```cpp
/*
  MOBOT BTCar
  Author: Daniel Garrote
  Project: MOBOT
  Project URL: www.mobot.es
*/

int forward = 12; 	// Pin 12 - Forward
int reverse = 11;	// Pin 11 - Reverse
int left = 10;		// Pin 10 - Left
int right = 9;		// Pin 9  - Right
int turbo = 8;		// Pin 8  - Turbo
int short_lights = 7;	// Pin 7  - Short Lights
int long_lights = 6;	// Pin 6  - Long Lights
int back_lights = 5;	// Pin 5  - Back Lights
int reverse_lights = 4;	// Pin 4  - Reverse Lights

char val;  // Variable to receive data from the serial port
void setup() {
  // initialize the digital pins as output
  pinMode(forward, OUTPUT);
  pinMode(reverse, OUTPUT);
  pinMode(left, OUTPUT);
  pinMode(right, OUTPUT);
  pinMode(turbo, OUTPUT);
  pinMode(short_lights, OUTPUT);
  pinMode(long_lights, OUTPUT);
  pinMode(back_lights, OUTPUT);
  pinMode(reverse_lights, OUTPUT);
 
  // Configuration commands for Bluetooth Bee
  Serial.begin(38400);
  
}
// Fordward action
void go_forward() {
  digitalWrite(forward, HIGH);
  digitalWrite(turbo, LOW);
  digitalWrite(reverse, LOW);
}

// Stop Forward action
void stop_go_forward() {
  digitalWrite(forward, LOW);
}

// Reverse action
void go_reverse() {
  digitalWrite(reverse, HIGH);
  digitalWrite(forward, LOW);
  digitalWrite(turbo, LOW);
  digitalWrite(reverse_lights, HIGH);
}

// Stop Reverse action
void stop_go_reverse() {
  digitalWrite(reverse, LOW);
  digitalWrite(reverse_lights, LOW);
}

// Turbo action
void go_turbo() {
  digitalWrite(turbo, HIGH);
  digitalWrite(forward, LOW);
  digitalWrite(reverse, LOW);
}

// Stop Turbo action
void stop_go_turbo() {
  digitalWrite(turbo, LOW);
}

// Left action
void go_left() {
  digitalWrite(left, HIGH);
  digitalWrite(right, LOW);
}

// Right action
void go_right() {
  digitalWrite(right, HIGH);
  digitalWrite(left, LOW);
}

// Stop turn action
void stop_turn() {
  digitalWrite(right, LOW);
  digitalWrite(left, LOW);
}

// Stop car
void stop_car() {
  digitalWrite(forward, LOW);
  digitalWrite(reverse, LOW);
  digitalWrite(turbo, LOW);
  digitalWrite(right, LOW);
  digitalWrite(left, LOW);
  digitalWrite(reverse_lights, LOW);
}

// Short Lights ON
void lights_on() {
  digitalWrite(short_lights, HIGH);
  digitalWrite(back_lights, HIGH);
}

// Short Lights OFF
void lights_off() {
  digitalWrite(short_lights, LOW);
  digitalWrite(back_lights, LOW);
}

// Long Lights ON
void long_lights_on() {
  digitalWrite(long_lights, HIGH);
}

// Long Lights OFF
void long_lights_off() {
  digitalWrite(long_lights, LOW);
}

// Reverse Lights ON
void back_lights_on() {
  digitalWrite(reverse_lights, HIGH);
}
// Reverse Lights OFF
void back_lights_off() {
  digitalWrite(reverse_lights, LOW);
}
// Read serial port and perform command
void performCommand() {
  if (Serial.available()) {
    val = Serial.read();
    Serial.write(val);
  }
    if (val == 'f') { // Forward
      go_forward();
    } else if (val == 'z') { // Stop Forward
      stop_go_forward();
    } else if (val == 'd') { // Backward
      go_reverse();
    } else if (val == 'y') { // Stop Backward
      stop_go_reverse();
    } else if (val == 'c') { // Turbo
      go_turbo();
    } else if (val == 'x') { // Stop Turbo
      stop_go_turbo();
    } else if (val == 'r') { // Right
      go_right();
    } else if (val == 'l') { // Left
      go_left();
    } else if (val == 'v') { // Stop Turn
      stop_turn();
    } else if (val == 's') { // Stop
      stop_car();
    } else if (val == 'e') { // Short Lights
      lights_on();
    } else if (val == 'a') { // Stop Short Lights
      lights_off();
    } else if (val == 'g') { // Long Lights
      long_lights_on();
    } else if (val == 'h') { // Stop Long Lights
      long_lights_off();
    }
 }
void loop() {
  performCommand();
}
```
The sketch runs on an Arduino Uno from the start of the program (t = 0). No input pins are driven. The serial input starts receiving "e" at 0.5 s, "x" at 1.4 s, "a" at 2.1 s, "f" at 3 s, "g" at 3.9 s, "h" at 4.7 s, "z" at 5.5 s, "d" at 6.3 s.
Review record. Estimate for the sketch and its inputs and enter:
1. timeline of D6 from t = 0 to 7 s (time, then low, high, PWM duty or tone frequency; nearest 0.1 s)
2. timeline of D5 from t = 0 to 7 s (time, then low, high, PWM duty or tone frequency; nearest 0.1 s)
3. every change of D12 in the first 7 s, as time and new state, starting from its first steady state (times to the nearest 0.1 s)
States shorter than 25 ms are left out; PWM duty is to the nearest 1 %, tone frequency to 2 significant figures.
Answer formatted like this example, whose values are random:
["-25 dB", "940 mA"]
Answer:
["0 s low; 3.9 s high; 4.7 s low", "0 s low; 0.5 s high; 2.1 s low", "0 s low; 3 s high; 5.5 s low"]
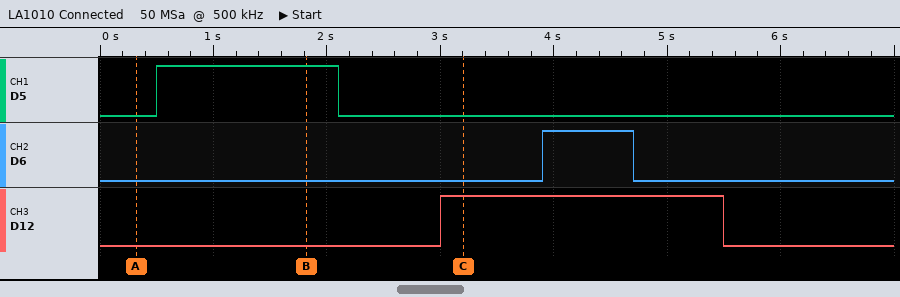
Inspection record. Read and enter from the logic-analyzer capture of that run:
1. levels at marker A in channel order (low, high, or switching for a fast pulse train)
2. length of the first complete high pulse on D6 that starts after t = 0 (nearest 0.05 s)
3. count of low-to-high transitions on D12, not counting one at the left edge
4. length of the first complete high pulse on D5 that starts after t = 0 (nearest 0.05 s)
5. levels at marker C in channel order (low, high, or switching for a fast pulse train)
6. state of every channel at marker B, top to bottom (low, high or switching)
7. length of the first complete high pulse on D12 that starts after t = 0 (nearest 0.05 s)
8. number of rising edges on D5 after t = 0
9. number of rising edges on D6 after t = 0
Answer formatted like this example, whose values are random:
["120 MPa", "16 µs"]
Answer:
["D5 low, D6 low, D12 low", "0.80 s", "1", "1.60 s", "D5 low, D6 low, D12 high", "D5 high, D6 low, D12 low", "2.50 s", "1", "1"]
